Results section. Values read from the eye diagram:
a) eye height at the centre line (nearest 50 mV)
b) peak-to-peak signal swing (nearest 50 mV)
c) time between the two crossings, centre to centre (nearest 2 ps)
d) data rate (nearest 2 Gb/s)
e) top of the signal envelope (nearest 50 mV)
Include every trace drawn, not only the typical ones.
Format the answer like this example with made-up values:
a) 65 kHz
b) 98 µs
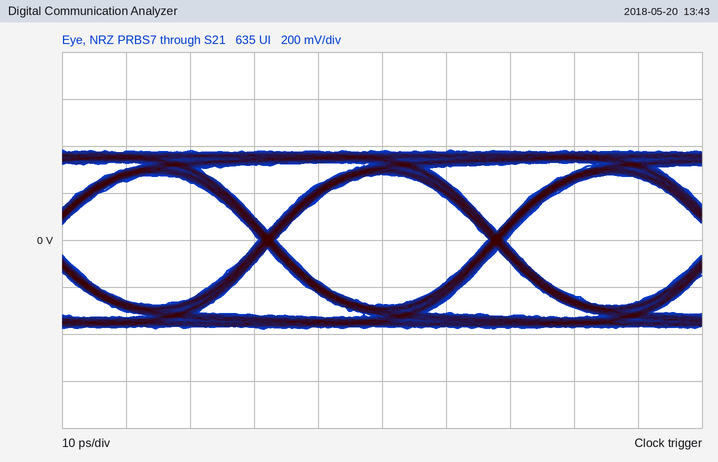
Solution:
a) 550 mV
b) 750 mV
c) 36 ps
d) 28 Gb/s
e) 400 mV
